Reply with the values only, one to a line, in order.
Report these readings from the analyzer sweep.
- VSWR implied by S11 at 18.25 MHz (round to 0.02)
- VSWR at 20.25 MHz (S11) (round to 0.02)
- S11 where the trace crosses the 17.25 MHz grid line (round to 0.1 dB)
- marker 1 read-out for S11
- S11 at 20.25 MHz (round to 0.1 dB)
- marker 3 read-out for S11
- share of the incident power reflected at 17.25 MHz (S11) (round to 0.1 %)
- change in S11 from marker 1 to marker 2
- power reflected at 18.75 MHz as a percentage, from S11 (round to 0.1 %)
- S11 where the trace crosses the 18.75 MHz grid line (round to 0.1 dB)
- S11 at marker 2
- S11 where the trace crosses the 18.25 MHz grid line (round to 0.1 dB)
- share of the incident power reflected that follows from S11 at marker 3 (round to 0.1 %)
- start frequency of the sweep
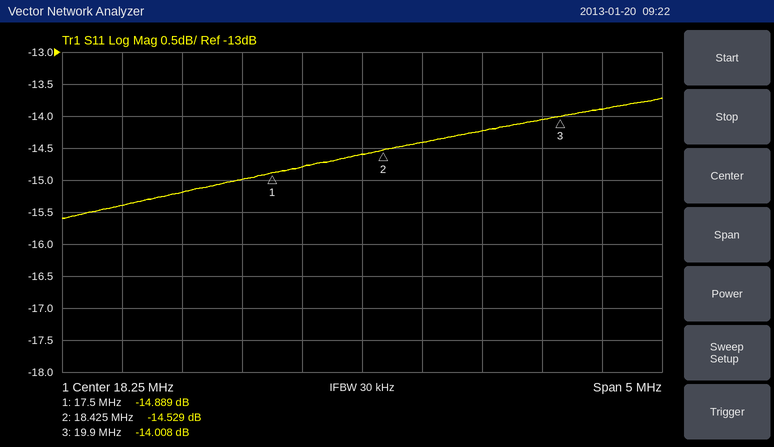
1.46
1.50
-15.0 dB
-14.889 dB
-13.9 dB
-14.008 dB
3.2 %
0.360 dB
3.6 %
-14.4 dB
-14.529 dB
-14.6 dB
4.0 %
15.75 MHz
